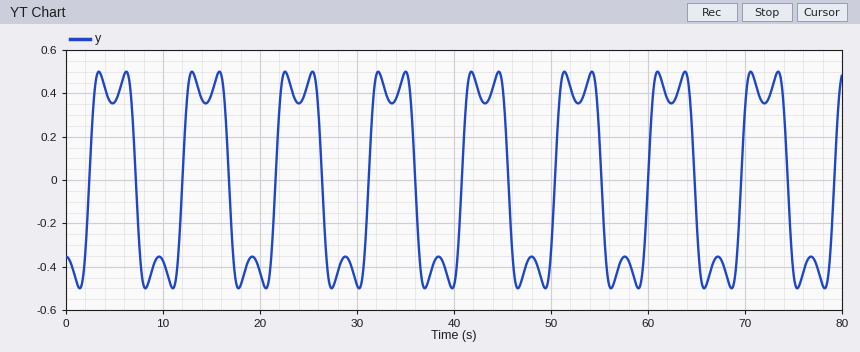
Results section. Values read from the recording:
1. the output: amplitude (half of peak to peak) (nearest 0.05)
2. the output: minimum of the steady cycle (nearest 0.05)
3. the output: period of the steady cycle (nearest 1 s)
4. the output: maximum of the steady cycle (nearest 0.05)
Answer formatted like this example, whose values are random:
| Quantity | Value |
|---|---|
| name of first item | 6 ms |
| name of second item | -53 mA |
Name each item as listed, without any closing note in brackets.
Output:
| Quantity | Value |
|---|---|
| the output: amplitude (half of peak to peak) | 0.50 |
| the output: minimum of the steady cycle | -0.50 |
| the output: period of the steady cycle | 10 s |
| the output: maximum of the steady cycle | 0.50 |
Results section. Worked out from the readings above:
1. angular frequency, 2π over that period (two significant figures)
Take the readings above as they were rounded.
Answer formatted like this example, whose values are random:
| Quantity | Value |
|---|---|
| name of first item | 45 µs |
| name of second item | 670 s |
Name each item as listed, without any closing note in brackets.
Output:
| Quantity | Value |
|---|---|
| angular frequency, 2π over that period | 0.63 rad/s |
